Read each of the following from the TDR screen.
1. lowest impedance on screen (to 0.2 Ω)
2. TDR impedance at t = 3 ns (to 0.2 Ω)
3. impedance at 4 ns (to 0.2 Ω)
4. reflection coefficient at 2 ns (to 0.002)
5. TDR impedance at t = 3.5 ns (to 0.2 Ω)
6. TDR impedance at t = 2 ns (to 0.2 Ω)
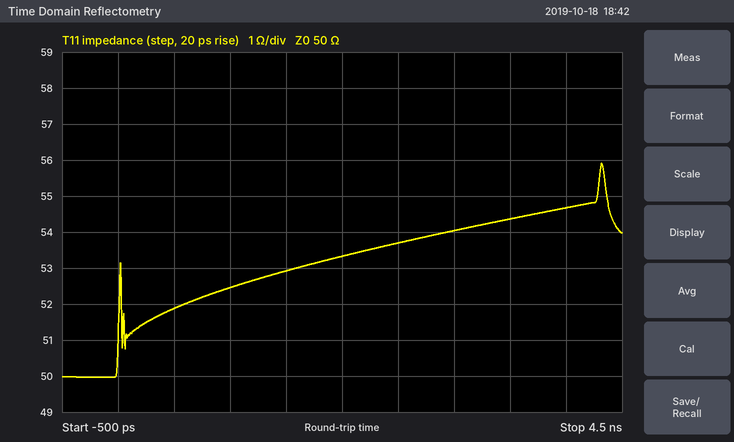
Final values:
50.0 Ω
54.0 Ω
54.6 Ω
+0.032
54.4 Ω
53.4 Ω
